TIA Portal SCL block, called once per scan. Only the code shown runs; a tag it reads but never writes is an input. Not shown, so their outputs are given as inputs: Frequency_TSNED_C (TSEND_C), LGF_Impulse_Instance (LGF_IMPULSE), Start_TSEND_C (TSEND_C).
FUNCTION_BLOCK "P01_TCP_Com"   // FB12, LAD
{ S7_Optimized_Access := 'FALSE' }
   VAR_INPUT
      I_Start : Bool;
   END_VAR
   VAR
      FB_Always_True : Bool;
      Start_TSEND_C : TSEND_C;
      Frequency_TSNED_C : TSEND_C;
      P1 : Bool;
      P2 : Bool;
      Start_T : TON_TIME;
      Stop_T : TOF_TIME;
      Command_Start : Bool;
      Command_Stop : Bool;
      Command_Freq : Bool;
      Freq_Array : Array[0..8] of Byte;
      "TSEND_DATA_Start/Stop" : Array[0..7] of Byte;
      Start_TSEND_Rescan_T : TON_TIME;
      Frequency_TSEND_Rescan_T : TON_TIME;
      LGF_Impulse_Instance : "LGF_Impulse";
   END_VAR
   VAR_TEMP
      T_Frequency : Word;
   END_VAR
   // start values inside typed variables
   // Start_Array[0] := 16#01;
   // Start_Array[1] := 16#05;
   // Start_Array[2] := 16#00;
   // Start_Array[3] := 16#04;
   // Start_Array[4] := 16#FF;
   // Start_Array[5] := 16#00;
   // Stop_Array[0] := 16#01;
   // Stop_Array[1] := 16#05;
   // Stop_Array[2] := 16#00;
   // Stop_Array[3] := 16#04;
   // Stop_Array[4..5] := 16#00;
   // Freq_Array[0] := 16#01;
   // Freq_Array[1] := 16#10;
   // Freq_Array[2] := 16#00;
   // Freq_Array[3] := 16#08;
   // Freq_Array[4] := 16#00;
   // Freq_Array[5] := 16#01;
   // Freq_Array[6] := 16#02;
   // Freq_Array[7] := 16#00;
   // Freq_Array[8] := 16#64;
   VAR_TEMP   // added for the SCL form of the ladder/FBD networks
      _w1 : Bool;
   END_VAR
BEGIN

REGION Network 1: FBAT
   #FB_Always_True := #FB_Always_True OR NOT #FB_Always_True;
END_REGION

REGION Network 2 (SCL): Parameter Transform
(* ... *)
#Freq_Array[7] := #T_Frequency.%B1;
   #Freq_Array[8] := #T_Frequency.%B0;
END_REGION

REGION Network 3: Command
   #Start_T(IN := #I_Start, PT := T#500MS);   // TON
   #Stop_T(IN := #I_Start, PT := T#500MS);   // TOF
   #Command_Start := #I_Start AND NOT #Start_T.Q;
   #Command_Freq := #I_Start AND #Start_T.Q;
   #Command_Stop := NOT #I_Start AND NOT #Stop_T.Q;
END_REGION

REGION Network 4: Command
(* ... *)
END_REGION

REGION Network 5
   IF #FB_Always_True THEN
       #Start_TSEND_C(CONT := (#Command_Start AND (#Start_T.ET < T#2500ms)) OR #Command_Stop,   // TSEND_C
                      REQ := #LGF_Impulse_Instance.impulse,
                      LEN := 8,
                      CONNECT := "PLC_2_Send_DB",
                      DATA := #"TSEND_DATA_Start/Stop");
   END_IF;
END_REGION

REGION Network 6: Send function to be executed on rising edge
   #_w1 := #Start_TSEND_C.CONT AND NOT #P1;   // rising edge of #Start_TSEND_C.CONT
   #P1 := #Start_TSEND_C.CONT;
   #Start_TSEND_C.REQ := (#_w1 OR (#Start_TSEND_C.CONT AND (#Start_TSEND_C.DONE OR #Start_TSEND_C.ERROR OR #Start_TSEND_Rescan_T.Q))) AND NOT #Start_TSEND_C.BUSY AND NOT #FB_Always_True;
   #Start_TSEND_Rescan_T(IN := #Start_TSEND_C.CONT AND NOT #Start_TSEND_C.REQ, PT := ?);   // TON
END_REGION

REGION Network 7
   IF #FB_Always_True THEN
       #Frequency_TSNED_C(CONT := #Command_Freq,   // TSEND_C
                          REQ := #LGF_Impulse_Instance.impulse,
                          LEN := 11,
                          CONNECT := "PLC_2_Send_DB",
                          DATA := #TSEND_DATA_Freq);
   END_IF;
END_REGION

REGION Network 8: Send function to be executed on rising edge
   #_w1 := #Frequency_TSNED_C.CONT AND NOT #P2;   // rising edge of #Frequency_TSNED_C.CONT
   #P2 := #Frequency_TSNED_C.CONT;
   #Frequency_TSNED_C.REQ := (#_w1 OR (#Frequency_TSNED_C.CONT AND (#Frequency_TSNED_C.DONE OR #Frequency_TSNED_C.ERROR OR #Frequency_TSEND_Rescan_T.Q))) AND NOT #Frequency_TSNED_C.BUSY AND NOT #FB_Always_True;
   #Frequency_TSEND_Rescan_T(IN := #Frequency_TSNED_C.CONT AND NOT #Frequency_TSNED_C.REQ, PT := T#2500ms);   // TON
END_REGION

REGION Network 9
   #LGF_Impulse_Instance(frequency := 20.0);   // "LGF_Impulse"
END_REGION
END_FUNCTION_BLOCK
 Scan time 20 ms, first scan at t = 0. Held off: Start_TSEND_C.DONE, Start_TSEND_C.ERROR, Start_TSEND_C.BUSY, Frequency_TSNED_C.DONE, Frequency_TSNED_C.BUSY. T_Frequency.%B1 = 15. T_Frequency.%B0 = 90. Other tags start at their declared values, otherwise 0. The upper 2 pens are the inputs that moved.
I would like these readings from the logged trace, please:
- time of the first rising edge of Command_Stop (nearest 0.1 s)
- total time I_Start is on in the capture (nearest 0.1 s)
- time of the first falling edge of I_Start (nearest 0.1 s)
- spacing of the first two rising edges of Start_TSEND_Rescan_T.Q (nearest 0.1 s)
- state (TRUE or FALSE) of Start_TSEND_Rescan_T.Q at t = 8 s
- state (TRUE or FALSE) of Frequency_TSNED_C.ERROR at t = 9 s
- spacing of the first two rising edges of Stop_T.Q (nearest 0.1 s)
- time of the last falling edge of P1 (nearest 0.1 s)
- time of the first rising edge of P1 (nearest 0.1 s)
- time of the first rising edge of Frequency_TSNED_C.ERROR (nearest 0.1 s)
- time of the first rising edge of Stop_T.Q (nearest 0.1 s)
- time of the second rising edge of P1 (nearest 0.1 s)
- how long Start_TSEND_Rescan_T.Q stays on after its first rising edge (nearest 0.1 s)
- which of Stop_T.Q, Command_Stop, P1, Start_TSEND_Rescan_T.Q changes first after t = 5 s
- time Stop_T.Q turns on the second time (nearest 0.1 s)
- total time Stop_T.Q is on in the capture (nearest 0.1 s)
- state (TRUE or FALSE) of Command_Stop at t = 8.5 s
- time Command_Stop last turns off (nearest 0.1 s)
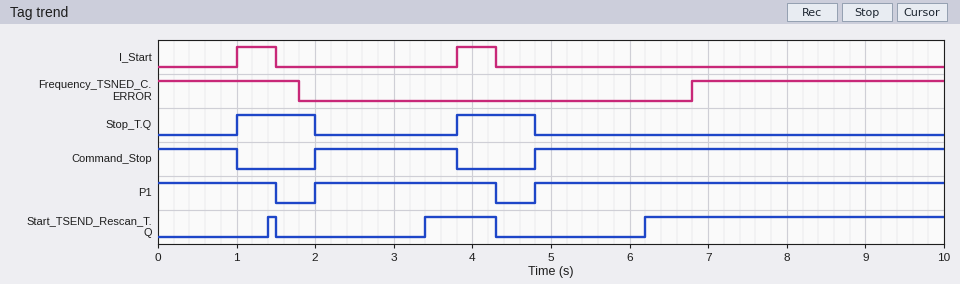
2.0 s
1.0 s
1.5 s
2.0 s
TRUE
TRUE
2.8 s
4.3 s
2.0 s
6.8 s
1.0 s
4.8 s
0.1 s
Start_TSEND_Rescan_T.Q
3.8 s
2.0 s
TRUE
3.8 s
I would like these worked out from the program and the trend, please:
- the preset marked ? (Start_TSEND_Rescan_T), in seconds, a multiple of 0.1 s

1.4 s
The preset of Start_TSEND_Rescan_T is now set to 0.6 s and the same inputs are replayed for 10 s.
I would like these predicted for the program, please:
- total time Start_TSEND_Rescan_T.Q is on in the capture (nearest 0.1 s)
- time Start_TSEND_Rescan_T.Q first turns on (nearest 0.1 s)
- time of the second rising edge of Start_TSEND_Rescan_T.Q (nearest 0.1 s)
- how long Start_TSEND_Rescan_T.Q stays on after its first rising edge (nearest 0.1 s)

7.2 s
0.6 s
2.6 s
0.9 s
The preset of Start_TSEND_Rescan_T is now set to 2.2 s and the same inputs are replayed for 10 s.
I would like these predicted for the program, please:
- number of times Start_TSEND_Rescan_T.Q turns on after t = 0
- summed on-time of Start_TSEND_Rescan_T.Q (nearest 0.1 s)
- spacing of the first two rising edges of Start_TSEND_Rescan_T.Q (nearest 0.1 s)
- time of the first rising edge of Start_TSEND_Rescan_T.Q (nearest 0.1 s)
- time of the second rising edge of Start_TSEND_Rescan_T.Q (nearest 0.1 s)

2
3.1 s
2.8 s
4.2 s
7.0 s
